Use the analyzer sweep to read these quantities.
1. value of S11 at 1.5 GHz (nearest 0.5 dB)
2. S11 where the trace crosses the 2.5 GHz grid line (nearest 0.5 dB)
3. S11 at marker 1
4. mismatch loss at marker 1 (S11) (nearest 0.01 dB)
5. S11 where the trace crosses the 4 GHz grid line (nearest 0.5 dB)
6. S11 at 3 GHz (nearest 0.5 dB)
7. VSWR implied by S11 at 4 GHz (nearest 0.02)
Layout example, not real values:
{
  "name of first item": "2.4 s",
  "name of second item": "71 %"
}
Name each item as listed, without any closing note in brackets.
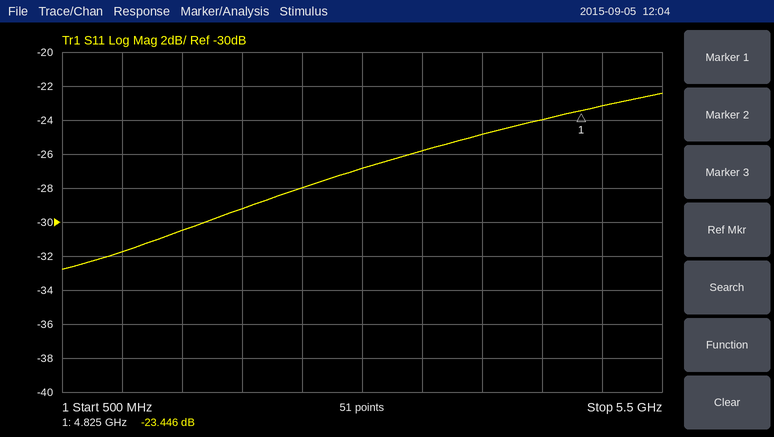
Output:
{
  "value of S11 at 1.5 GHz": "-30.5 dB",
  "S11 where the trace crosses the 2.5 GHz grid line": "-28.0 dB",
  "S11 at marker 1": "-23.446 dB",
  "mismatch loss at marker 1 (S11)": "0.02 dB",
  "S11 where the trace crosses the 4 GHz grid line": "-25.0 dB",
  "S11 at 3 GHz": "-27.0 dB",
  "VSWR implied by S11 at 4 GHz": "1.12"
}
